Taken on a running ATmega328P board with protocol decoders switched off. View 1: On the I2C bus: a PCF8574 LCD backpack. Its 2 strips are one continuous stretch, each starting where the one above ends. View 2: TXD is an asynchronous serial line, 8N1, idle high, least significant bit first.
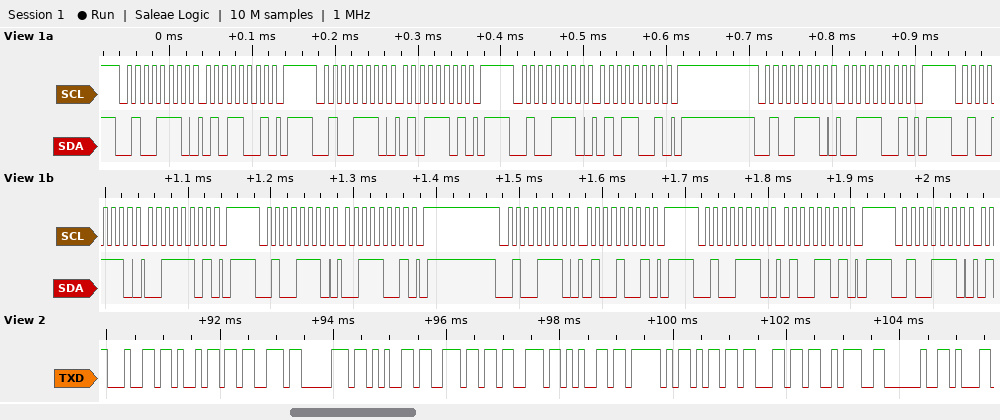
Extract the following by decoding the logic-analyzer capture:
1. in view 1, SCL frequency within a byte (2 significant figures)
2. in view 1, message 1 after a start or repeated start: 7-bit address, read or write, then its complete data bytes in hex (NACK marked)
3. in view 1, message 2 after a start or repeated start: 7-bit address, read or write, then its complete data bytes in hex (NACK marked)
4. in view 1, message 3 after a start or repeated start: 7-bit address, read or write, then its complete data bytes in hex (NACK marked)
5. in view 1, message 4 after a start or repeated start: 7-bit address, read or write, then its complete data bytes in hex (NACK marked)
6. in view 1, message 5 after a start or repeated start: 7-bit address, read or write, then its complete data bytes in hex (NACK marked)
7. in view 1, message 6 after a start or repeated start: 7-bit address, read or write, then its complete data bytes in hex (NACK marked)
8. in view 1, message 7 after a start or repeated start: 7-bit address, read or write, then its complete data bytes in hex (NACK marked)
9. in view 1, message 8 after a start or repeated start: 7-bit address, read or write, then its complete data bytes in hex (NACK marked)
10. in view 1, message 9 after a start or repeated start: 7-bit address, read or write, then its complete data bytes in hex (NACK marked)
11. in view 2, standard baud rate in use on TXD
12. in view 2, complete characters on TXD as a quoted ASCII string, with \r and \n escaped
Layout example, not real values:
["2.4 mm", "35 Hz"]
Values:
["100 kHz", "0x27 write: 59", "0x27 write: 5D", "0x27 write: 59", "0x27 write: 39", "0x27 write: 3D", "0x27 write: 39", "0x27 write: 49", "0x27 write: 4D", "0x27 write", "9600 baud", "\"dispense_ml: \""]
